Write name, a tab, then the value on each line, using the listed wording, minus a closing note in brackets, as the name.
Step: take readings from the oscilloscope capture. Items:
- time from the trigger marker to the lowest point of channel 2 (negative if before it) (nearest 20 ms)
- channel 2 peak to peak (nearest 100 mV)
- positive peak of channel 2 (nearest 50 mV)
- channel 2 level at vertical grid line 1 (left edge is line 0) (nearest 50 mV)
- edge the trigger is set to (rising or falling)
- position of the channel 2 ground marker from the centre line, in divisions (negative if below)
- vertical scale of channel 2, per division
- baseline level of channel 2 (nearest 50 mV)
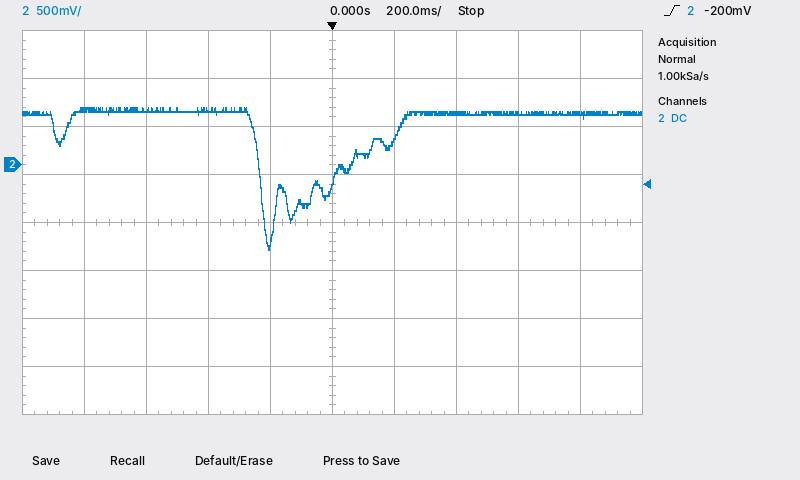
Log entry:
time from the trigger marker to the lowest point of channel 2 (negative if before it)	-200 ms
channel 2 peak to peak	1.50 V
positive peak of channel 2	600 mV
channel 2 level at vertical grid line 1 (left edge is line 0)	600 mV
edge the trigger is set to	rising
position of the channel 2 ground marker from the centre line, in divisions	+1.2 div
vertical scale of channel 2, per division	500 mV
baseline level of channel 2	550 mV
